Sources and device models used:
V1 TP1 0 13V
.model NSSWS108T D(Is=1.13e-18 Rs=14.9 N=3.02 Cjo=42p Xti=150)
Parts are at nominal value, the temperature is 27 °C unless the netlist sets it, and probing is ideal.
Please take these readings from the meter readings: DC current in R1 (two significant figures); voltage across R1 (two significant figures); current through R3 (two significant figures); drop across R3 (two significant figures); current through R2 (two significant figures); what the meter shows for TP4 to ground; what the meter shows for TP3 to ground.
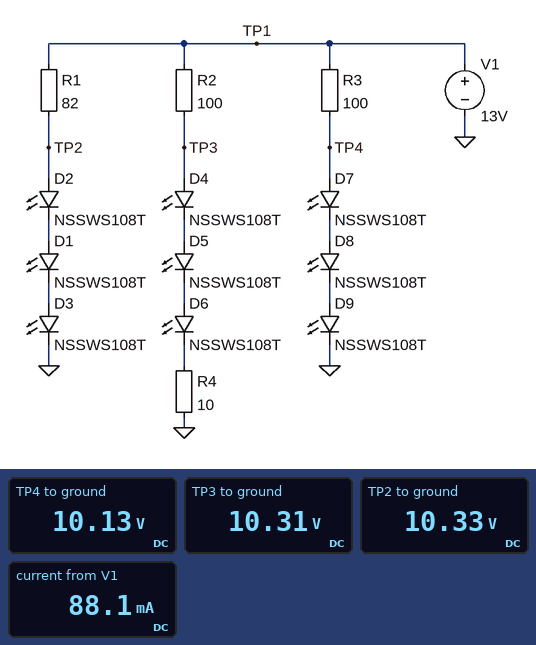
33 mA
2.7 V
29 mA
2.9 V
27 mA
10.13 V
10.31 V
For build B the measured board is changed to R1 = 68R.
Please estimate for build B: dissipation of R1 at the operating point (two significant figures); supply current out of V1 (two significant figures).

90 mW
92 mA
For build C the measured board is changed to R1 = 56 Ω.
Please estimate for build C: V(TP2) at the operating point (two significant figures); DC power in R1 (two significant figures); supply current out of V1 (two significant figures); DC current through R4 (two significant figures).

11 V
91 mW
96 mA
27 mA
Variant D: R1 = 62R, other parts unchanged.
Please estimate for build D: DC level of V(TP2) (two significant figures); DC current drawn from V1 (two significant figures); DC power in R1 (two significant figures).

11 V
94 mA
91 mW
